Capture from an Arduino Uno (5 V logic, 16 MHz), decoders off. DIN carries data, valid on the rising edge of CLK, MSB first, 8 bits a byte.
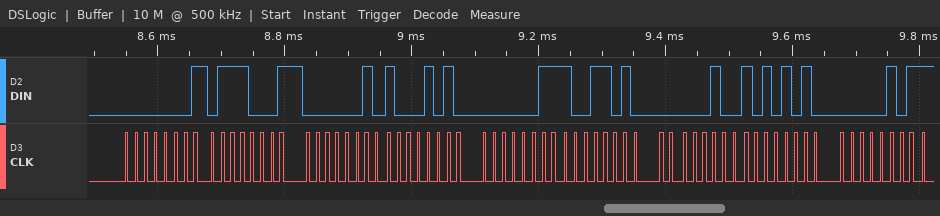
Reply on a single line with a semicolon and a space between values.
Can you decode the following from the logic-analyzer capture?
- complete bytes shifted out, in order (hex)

01 71 02 8A 03 9A 04 AA 05
